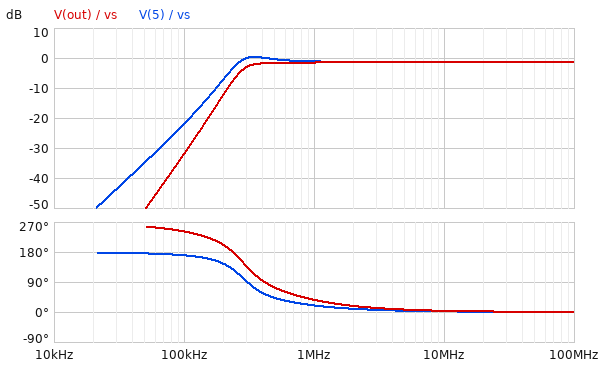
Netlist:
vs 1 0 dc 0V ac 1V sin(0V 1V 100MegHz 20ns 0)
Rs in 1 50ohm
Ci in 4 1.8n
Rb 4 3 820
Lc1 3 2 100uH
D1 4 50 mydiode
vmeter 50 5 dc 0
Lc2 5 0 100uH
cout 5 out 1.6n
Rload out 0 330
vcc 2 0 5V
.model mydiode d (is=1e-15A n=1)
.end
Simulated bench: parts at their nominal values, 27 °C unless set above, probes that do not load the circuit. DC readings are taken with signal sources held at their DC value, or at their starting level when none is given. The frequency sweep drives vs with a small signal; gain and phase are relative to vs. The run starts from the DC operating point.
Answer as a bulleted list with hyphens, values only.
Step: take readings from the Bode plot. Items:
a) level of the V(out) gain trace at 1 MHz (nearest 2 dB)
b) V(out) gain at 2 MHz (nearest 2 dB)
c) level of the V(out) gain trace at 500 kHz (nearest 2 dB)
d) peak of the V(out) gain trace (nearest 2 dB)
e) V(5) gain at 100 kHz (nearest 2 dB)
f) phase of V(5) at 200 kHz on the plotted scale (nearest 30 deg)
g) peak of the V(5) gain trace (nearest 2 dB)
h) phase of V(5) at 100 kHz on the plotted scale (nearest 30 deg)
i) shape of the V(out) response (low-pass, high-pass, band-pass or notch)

- -2 dB
- -2 dB
- -2 dB
- -2 dB
- -22 dB
- 150 deg
- 0 dB
- 180 deg
- high-pass
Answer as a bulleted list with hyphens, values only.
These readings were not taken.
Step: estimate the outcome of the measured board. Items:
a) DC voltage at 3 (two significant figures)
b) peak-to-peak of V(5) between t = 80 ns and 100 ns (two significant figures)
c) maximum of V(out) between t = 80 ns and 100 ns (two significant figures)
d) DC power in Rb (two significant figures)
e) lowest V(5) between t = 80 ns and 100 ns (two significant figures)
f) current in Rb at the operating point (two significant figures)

- 5.0 V
- 1.7 V
- 850 mV
- 22 mW
- -860 mV
- 5.2 mA
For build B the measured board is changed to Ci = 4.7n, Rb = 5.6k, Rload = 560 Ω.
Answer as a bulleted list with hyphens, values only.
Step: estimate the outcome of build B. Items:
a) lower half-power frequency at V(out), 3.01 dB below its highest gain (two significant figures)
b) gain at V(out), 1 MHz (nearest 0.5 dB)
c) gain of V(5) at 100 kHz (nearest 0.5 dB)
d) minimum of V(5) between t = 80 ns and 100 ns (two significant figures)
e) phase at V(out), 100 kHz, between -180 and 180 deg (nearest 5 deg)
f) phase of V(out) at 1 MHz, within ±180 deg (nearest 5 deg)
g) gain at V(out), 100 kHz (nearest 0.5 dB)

- 180 kHz
- -1.0 dB
- -13.0 dB
- -470 mV
- -140 deg
- 20 deg
- -19.0 dB
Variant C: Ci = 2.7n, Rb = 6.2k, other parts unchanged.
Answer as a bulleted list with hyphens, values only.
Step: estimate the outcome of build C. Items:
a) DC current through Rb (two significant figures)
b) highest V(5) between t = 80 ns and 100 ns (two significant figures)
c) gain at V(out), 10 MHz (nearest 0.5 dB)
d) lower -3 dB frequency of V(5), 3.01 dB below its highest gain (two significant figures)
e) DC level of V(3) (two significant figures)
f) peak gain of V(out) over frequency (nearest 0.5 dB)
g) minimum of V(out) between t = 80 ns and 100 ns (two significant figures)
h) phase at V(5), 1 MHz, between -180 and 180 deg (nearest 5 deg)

- 690 µA
- 820 mV
- -2.0 dB
- 210 kHz
- 5.0 V
- -0.5 dB
- -270 mV
- 10 deg
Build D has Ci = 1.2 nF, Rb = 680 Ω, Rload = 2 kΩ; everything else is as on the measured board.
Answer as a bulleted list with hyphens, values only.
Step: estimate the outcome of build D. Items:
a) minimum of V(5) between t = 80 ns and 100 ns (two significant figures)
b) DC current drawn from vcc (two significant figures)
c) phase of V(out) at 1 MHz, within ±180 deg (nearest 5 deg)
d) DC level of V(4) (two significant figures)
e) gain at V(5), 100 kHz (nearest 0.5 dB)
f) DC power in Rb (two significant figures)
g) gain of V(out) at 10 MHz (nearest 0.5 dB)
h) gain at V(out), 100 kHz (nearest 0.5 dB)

- -980 mV
- 6.2 mA
- 25 deg
- 760 mV
- -26.0 dB
- 26 mW
- 0 dB
- -27.0 dB
